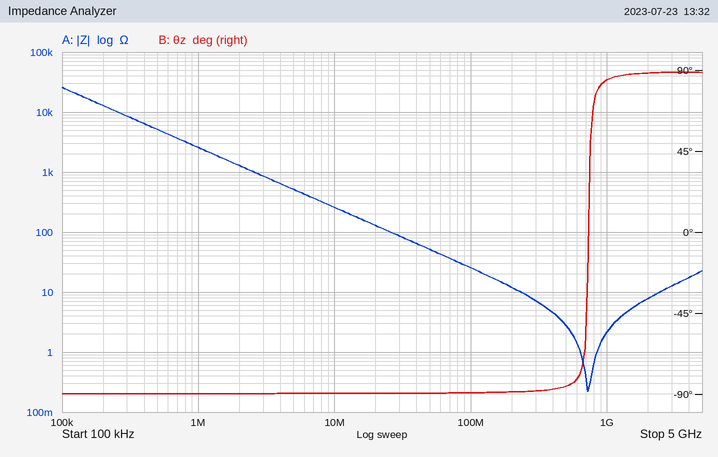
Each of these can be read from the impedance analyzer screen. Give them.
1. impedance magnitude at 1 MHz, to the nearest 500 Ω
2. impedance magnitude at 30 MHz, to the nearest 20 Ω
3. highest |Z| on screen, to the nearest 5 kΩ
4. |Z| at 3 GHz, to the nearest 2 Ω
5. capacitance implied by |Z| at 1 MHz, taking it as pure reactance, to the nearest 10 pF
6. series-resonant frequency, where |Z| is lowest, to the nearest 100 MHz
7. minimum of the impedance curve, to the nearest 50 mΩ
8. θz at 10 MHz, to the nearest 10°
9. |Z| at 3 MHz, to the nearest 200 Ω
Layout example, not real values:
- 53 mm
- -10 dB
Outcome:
- 2.5 kΩ
- 80 Ω
- 25 kΩ
- 12 Ω
- 60 pF
- 700 MHz
- 200 mΩ
- -90°
- 800 Ω
